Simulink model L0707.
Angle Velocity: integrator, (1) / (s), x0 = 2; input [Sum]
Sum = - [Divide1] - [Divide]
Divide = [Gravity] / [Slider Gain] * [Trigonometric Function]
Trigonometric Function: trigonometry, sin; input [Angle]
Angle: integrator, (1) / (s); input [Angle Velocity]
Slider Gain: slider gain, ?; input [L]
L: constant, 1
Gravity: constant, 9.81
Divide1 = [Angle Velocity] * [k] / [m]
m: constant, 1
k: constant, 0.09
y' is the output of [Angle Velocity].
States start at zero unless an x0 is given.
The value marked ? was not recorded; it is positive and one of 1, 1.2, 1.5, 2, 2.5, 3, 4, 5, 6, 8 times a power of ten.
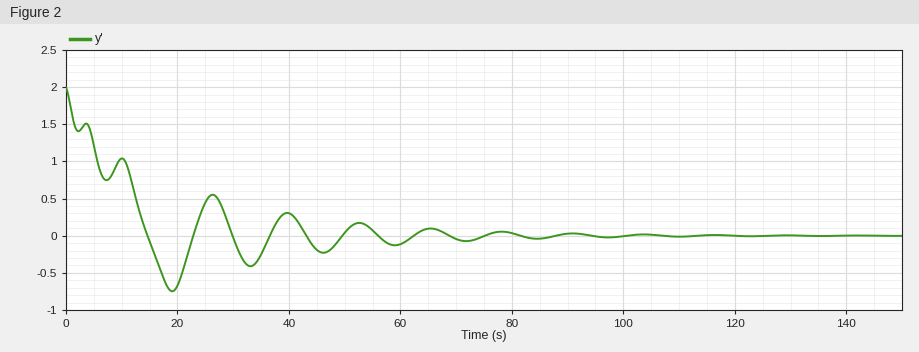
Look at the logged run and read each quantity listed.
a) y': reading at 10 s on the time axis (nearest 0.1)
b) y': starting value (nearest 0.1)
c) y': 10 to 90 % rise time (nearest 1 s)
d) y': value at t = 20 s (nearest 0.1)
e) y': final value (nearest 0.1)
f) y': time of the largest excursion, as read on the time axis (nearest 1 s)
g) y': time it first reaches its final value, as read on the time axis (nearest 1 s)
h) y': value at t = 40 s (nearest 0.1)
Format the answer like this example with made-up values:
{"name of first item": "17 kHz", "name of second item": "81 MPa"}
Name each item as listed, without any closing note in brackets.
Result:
{"y': reading at 10 s on the time axis": "1.0", "y': starting value": "2.0", "y': 10 to 90 % rise time": "13 s", "y': value at t = 20 s": "-0.7", "y': final value": "0.0", "y': time of the largest excursion, as read on the time axis": "19 s", "y': time it first reaches its final value, as read on the time axis": "15 s", "y': value at t = 40 s": "0.3"}
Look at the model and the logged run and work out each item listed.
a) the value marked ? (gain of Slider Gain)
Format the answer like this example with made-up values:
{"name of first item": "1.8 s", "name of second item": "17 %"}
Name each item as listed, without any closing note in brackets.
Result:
{"the value marked ?": "40"}
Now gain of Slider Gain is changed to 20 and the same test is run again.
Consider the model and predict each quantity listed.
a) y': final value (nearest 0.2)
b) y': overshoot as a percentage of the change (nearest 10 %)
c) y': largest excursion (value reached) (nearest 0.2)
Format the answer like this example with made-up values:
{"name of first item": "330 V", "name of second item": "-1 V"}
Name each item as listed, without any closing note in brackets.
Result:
{"y': final value": "0.0", "y': overshoot as a percentage of the change": "60 %", "y': largest excursion (value reached)": "-1.2"}
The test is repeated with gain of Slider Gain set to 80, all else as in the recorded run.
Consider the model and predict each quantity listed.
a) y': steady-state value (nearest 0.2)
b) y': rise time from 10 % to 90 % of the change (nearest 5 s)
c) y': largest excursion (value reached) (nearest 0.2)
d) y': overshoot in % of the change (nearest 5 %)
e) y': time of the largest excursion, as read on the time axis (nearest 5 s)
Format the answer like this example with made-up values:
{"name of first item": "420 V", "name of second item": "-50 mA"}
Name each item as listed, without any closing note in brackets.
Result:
{"y': steady-state value": "0.0", "y': rise time from 10 % to 90 % of the change": "25 s", "y': largest excursion (value reached)": "-0.4", "y': overshoot in % of the change": "20 %", "y': time of the largest excursion, as read on the time axis": "35 s"}
